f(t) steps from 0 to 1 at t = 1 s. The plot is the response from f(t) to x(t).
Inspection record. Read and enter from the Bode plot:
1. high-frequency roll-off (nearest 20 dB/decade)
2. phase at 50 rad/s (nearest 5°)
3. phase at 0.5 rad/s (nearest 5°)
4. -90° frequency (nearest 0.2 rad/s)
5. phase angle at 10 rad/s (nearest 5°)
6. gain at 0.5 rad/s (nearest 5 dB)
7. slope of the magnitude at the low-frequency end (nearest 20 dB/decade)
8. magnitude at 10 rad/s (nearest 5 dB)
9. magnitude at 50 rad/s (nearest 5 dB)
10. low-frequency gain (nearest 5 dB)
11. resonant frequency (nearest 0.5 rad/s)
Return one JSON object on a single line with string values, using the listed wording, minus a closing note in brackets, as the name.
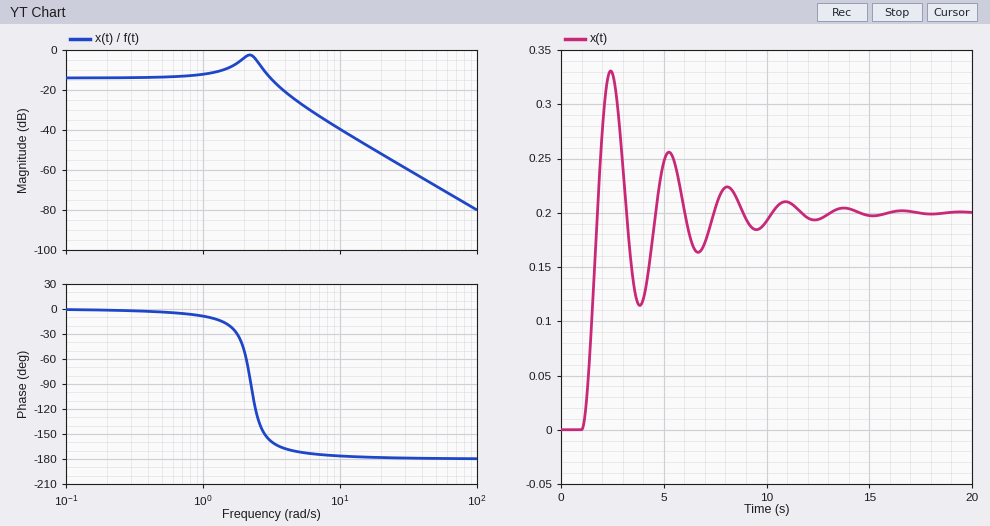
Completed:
{"high-frequency roll-off": "-40 dB/decade", "phase at 50 rad/s": "-180°", "phase at 0.5 rad/s": "-5°", "-90° frequency": "2.2 rad/s", "phase angle at 10 rad/s": "-175°", "gain at 0.5 rad/s": "-15 dB", "slope of the magnitude at the low-frequency end": "0 dB/decade", "magnitude at 10 rad/s": "-40 dB", "magnitude at 50 rad/s": "-70 dB", "low-frequency gain": "-15 dB", "resonant frequency": "2.0 rad/s"}
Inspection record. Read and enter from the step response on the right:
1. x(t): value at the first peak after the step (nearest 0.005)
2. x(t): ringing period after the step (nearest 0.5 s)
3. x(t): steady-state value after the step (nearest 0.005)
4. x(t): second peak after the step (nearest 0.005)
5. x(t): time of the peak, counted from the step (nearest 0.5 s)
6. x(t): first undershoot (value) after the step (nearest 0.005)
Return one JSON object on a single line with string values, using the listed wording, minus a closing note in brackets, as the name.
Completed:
{"x(t): value at the first peak after the step": "0.330", "x(t): ringing period after the step": "3.0 s", "x(t): steady-state value after the step": "0.200", "x(t): second peak after the step": "0.255", "x(t): time of the peak, counted from the step": "1.5 s", "x(t): first undershoot (value) after the step": "0.115"}
